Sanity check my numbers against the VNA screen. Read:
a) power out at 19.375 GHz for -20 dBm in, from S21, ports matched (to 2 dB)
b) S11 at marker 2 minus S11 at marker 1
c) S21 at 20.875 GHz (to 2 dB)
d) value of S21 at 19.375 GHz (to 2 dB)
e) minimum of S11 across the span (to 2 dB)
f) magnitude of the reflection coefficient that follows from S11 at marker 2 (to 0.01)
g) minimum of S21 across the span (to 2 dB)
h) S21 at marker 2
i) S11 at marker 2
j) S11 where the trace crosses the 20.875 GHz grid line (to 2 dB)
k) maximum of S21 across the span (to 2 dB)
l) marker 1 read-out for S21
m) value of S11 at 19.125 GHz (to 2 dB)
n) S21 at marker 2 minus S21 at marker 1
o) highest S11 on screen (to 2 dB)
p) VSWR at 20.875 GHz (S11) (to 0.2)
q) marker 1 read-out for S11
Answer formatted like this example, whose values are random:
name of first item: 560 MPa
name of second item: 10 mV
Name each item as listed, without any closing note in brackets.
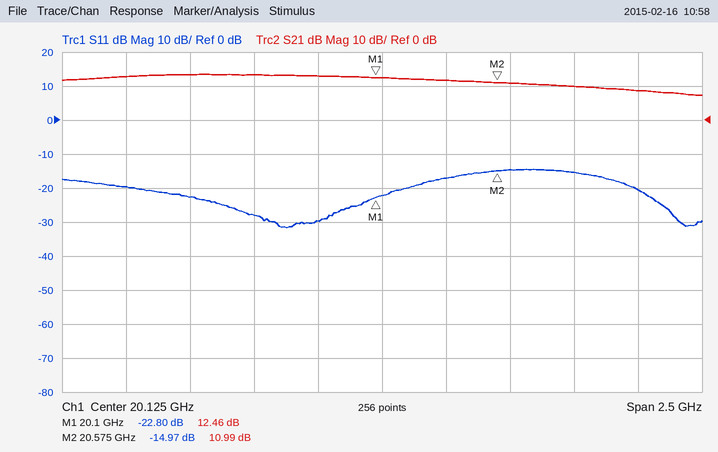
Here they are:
power out at 19.375 GHz for -20 dBm in, from S21, ports matched: -6 dBm
S11 at marker 2 minus S11 at marker 1: 7.83 dB
S21 at 20.875 GHz: 10 dB
value of S21 at 19.375 GHz: 14 dB
minimum of S11 across the span: -32 dB
magnitude of the reflection coefficient that follows from S11 at marker 2: 0.18
minimum of S21 across the span: 8 dB
S21 at marker 2: 10.99 dB
S11 at marker 2: -14.97 dB
S11 where the trace crosses the 20.875 GHz grid line: -16 dB
maximum of S21 across the span: 14 dB
marker 1 read-out for S21: 12.46 dB
value of S11 at 19.125 GHz: -20 dB
S21 at marker 2 minus S21 at marker 1: -1.47 dB
highest S11 on screen: -14 dB
VSWR at 20.875 GHz (S11): 1.4
marker 1 read-out for S11: -22.80 dB
